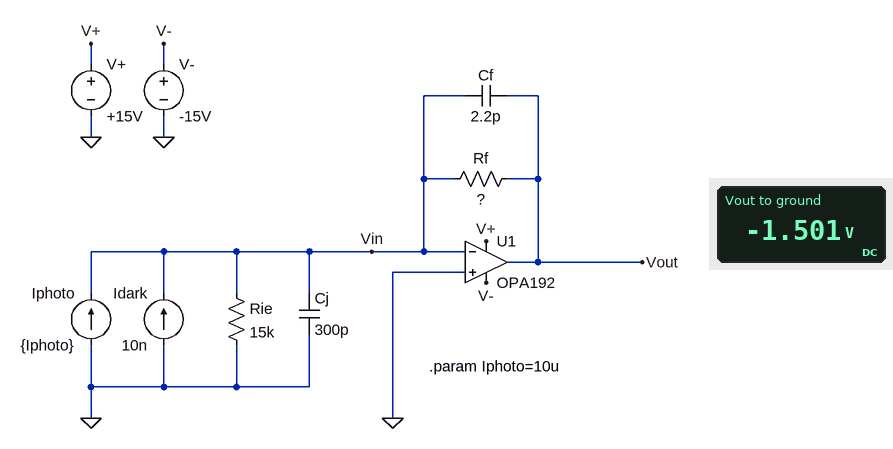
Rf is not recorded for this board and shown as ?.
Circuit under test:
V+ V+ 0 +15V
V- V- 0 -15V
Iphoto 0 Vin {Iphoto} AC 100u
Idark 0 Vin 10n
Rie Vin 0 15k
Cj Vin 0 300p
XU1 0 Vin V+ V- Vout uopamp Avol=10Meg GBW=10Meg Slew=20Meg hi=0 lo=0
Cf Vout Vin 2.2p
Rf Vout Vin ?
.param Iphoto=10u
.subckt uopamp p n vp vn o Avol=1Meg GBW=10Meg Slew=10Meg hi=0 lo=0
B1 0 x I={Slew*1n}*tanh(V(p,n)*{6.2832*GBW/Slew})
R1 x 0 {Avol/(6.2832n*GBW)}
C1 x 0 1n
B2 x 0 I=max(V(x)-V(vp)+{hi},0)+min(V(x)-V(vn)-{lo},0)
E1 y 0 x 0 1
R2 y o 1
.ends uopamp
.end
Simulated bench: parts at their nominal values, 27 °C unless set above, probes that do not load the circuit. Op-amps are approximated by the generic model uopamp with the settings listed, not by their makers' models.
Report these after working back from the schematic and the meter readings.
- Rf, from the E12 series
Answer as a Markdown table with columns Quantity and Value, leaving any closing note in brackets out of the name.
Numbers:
| Quantity | Value |
|---|---|
| Rf, from the E12 series | 150 kΩ |
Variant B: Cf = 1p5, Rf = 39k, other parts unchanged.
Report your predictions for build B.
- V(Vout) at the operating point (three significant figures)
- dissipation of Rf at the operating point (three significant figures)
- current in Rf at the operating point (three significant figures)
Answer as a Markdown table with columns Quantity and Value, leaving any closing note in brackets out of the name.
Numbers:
| Quantity | Value |
|---|---|
| V(Vout) at the operating point | -390 mV |
| dissipation of Rf at the operating point | 3.91 µW |
| current in Rf at the operating point | 10.0 µA |
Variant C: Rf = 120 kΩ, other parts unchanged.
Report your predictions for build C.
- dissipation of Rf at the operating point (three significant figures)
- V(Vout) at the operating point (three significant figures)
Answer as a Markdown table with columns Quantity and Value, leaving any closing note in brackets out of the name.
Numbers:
| Quantity | Value |
|---|---|
| dissipation of Rf at the operating point | 12.0 µW |
| V(Vout) at the operating point | -1.20 V |
